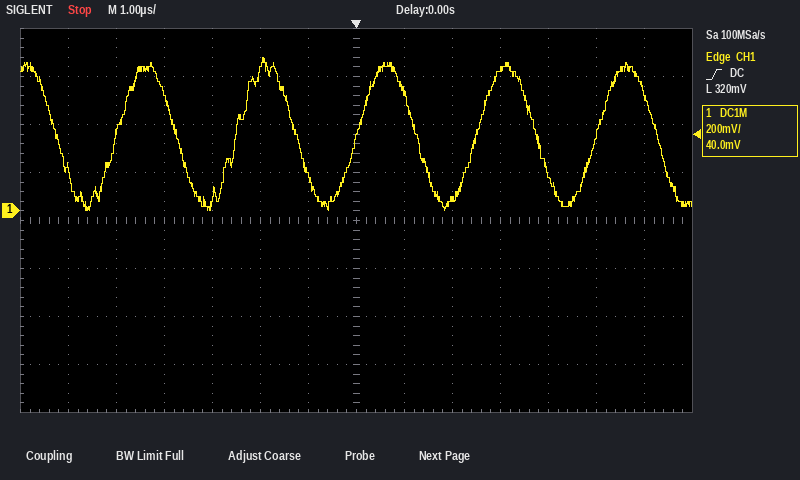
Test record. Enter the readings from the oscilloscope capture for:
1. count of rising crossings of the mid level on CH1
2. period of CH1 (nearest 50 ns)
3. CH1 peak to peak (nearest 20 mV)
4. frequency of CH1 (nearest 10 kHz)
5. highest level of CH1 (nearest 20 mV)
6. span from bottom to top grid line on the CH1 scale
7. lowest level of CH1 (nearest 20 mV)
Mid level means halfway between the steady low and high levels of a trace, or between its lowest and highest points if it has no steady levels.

5
2.50 µs
640 mV
400 kHz
640 mV
1.6 V
0 mV
